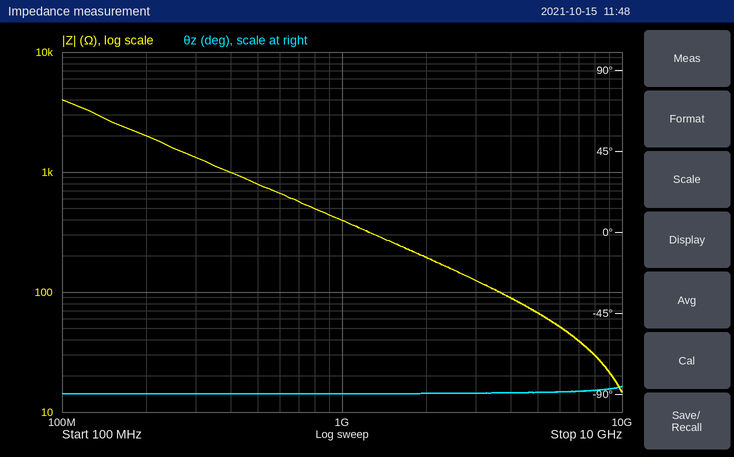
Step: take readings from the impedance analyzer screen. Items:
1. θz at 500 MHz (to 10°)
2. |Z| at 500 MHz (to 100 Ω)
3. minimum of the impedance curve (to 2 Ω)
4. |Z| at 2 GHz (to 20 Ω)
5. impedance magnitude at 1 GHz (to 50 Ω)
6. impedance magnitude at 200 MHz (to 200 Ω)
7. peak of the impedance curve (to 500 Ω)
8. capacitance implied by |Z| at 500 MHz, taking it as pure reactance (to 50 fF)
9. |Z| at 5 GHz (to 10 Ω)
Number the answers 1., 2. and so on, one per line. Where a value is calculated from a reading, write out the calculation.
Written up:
1. -90°
2. 800 Ω
3. 14 Ω
4. 200 Ω
5. 400 Ω
6. 2.0 kΩ
7. 4.0 kΩ
8. C = 1/(2π × 500 MHz × 800 Ω) ≈ 398 fF, so 400 fF to the nearest 50 fF
9. 70 Ω
